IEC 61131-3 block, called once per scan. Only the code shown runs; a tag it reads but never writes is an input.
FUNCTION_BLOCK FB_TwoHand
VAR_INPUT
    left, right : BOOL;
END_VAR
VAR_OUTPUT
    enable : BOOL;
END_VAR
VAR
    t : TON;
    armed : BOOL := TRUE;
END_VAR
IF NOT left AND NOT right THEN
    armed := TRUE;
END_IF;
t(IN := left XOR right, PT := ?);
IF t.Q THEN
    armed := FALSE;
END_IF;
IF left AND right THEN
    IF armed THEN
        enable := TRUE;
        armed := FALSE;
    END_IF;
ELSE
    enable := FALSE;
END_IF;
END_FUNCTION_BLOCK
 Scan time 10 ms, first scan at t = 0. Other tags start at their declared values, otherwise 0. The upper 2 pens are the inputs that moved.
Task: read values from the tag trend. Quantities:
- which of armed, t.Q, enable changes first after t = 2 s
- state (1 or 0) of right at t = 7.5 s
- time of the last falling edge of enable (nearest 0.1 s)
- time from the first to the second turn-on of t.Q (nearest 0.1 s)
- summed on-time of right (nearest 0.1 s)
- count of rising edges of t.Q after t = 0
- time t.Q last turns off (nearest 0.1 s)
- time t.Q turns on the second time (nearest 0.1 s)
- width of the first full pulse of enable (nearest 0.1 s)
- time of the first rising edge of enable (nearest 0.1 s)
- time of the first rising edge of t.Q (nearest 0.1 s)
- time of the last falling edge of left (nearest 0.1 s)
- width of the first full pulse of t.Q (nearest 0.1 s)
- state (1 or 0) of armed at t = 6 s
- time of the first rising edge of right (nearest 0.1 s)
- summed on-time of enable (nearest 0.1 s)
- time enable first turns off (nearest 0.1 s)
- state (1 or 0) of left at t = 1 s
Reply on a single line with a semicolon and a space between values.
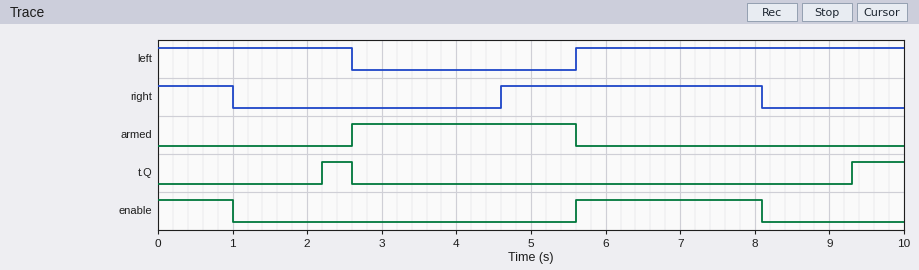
t.Q; 1; 8.1 s; 7.1 s; 4.5 s; 2; 2.6 s; 9.3 s; 2.5 s; 5.6 s; 2.2 s; 2.6 s; 0.4 s; 0; 4.6 s; 3.5 s; 1.0 s; 1
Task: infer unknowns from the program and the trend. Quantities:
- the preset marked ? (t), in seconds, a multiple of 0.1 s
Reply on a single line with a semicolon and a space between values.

1.2 s
